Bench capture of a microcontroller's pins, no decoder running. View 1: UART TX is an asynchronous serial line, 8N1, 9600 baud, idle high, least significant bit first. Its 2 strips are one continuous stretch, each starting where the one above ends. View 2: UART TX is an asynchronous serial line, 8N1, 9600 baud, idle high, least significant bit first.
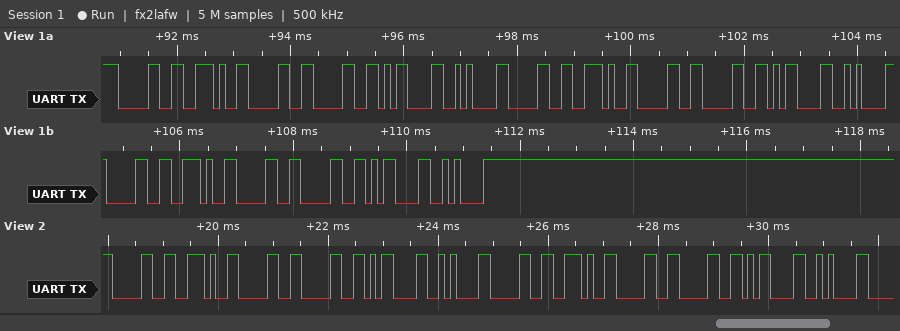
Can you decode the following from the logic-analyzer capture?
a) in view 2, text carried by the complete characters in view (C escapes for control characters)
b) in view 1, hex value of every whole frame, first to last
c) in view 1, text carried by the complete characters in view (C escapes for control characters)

"0.00\r\n0.00\r\n"
0x30 0x2E 0x30 0x30 0x0D 0x0A 0x30 0x2E 0x30 0x30 0x0D 0x0A 0x30 0x2E 0x30 0x30 0x0D 0x0A
"0.00\r\n0.00\r\n0.00\r\n"
